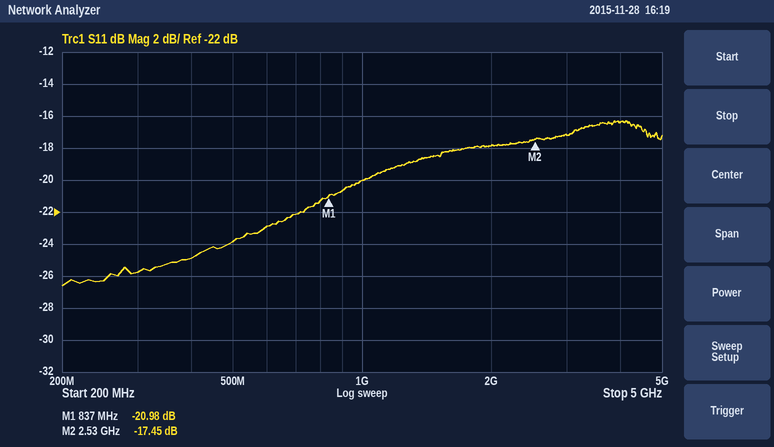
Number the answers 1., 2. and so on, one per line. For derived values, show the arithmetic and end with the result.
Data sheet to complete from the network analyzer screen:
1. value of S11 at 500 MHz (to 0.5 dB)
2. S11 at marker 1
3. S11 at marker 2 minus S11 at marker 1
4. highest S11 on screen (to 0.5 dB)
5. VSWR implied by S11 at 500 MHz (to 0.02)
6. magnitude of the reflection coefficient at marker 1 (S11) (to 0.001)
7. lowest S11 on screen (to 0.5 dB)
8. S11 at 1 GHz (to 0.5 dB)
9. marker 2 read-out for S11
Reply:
1. -24.0 dB
2. -20.98 dB
3. -17.45 − (-20.98) = 3.53 dB
4. -16.5 dB
5. |Γ| = 10^(-24/20) = 0.0631; VSWR = (1 + 0.0631)/(1 − 0.0631) ≈ 1.13, so 1.14 to the nearest 0.02
6. 10^(-20.98/20) ≈ 0.089
7. -26.5 dB
8. -20.0 dB
9. -17.45 dB
